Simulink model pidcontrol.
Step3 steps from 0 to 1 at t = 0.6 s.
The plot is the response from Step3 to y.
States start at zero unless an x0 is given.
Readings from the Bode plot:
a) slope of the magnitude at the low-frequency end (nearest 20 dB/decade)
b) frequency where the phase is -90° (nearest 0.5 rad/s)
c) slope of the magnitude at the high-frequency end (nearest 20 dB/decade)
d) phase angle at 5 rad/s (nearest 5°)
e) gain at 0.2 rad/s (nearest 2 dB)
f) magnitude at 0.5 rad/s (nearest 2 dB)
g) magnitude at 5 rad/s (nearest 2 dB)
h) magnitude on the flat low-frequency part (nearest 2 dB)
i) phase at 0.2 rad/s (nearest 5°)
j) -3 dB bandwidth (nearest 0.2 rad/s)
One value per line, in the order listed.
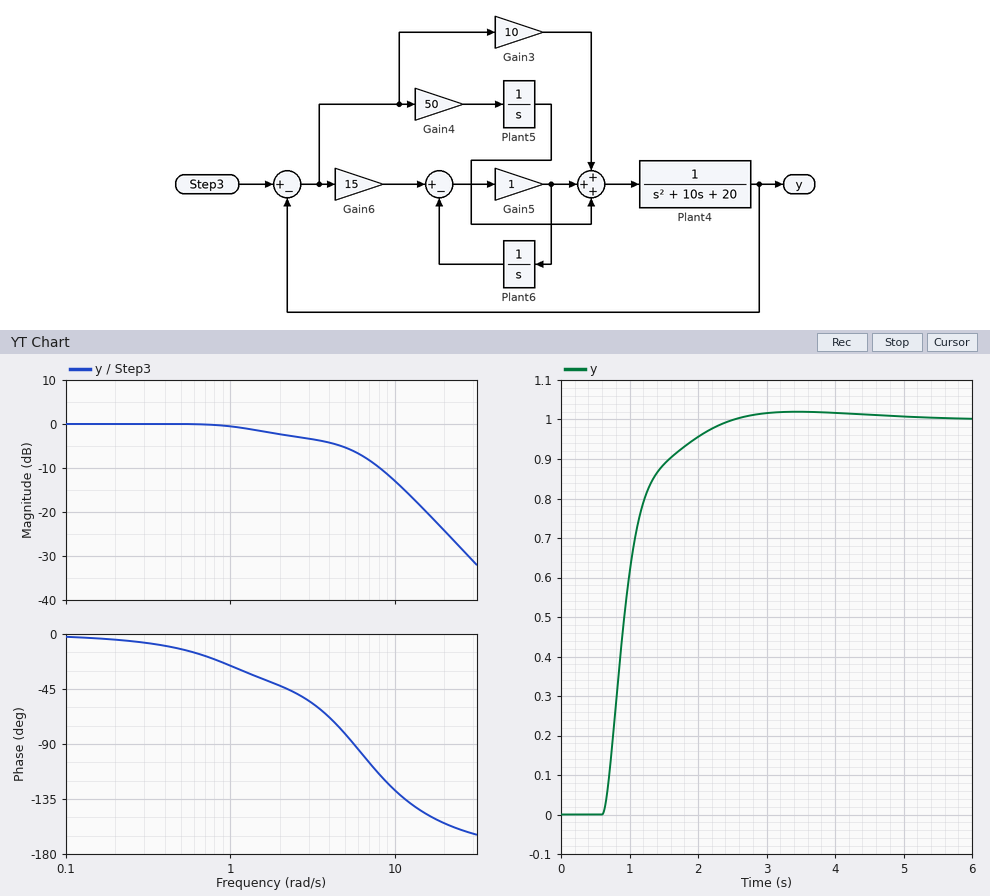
0 dB/decade
5.5 rad/s
-40 dB/decade
-80°
0 dB
0 dB
-6 dB
0 dB
-5°
2.6 rad/s
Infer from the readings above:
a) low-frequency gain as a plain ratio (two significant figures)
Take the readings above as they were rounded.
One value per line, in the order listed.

1.0
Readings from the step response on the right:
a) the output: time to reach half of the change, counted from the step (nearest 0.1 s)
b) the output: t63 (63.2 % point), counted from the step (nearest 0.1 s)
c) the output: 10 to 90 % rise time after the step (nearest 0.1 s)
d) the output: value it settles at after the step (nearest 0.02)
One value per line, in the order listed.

0.3 s
0.4 s
0.9 s
1.00
